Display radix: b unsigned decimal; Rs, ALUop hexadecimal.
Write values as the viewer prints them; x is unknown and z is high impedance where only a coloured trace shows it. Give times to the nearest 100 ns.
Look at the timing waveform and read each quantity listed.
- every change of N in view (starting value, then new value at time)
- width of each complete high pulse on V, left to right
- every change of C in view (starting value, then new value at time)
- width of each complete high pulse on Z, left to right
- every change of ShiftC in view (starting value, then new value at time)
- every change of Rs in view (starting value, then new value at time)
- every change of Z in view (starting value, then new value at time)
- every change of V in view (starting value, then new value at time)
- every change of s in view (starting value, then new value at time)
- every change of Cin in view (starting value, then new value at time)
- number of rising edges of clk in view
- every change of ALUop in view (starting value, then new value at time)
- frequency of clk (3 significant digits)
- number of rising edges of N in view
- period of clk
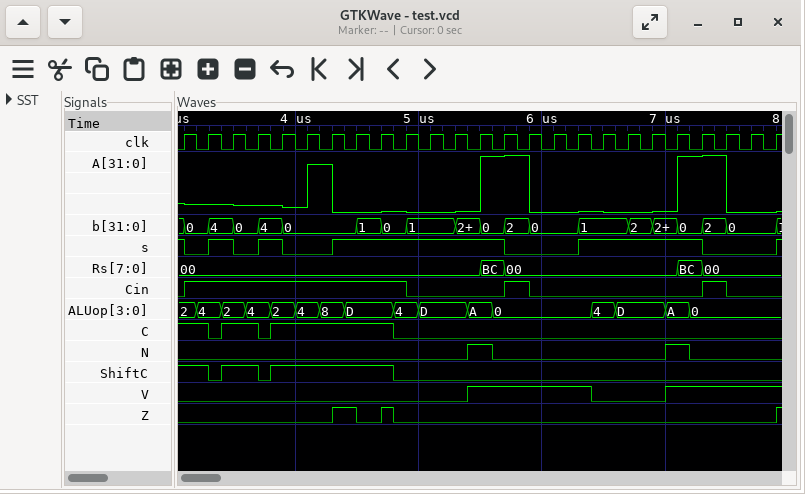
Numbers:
0, 1 at 5400 ns, 0 at 5600 ns, 1 at 7000 ns, 0 at 7200 ns
1000 ns
1, 0 at 3300 ns, 1 at 3400 ns, 0 at 3700 ns, 1 at 3800 ns, 0 at 4800 ns
200 ns, 100 ns
1, 0 at 3300 ns, 1 at 3400 ns, 0 at 3700 ns, 1 at 3800 ns, 0 at 4800 ns
00, BC at 5500 ns, 00 at 5700 ns, BC at 7100 ns, 00 at 7300 ns
0, 1 at 4300 ns, 0 at 4500 ns, 1 at 4700 ns, 0 at 4800 ns, 1 at 7900 ns
0, 1 at 5400 ns, 0 at 6400 ns, 1 at 7000 ns
1, 0 at 3100 ns, 1 at 3300 ns, 0 at 3500 ns, 1 at 3700 ns, 0 at 3900 ns, 1 at 4300 ns, 0 at 5700 ns, 1 at 6300 ns, 0 at 7300 ns, 1 at 7900 ns
0, 1 at 3100 ns, 0 at 4900 ns, 1 at 5700 ns, 0 at 5900 ns, 1 at 7300 ns, 0 at 7500 ns
25
2, 4 at 3200 ns, 2 at 3400 ns, 4 at 3600 ns, 2 at 3800 ns, 4 at 4000 ns, 8 at 4200 ns, D at 4400 ns, 4 at 4800 ns, D at 5000 ns, A at 5400 ns, 0 at 5600 ns, 4 at 6400 ns, D at 6600 ns, A at 7000 ns, 0 at 7200 ns
5.00 MHz
2
200 ns
